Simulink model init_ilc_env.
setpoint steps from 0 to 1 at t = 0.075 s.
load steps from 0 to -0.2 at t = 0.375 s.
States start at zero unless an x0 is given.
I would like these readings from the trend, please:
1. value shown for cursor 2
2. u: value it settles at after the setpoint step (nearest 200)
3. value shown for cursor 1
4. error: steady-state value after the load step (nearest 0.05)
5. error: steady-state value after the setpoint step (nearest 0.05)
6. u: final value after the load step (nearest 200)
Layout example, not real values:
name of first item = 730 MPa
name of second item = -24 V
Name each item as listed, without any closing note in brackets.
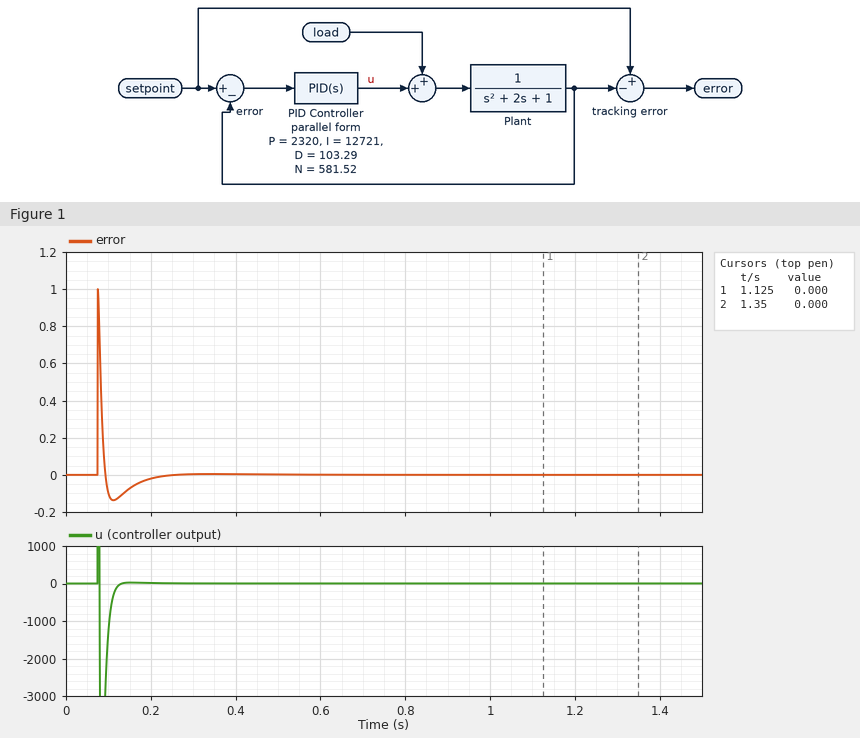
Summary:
value shown for cursor 2 = 0.000
u: value it settles at after the setpoint step = 0
value shown for cursor 1 = 0.000
error: steady-state value after the load step = 0.00
error: steady-state value after the setpoint step = 0.00
u: final value after the load step = 0
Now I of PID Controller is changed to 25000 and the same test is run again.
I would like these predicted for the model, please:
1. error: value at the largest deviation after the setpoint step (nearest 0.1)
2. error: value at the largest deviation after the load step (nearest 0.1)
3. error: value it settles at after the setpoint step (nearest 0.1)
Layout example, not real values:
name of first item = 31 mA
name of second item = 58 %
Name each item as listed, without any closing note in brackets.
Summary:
error: value at the largest deviation after the setpoint step = 1.0
error: value at the largest deviation after the load step = 0.0
error: value it settles at after the setpoint step = 0.0
